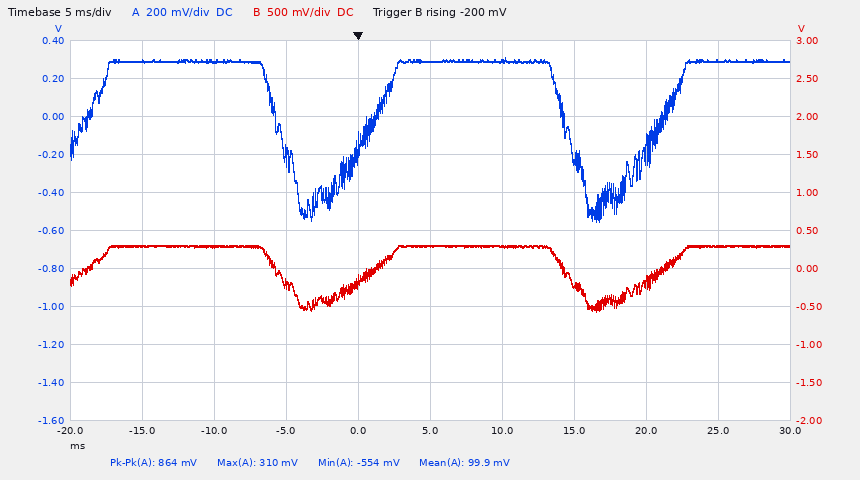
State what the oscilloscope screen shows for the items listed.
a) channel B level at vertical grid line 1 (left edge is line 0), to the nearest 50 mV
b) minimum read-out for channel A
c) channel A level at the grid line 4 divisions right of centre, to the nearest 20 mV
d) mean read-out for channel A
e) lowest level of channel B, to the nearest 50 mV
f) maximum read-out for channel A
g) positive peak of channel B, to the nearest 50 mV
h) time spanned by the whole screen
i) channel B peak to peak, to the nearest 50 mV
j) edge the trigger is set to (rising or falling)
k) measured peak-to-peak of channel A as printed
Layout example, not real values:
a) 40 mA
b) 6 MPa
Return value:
a) 300 mV
b) -554 mV
c) 300 mV
d) 99.9 mV
e) -550 mV
f) 310 mV
g) 300 mV
h) 50 ms
i) 850 mV
j) rising
k) 864 mV
